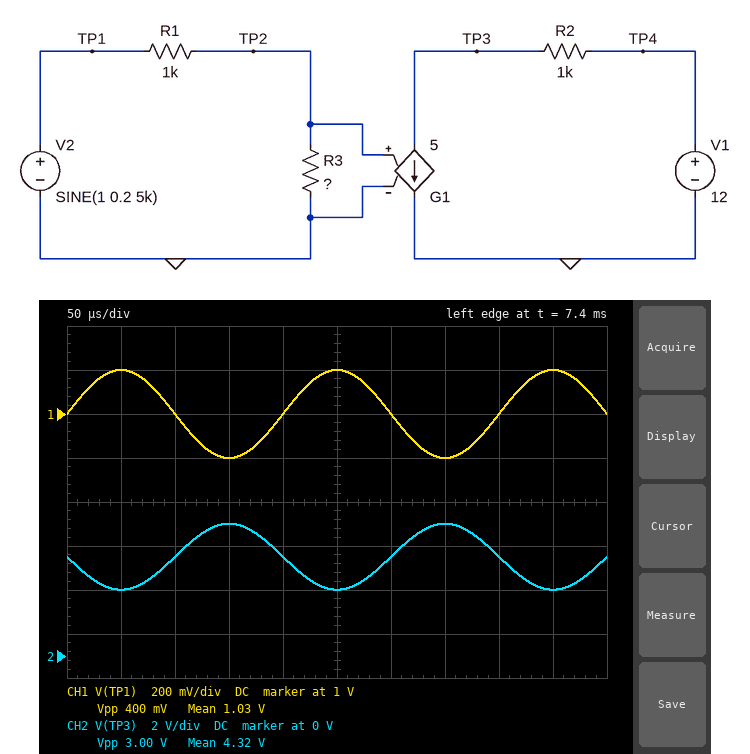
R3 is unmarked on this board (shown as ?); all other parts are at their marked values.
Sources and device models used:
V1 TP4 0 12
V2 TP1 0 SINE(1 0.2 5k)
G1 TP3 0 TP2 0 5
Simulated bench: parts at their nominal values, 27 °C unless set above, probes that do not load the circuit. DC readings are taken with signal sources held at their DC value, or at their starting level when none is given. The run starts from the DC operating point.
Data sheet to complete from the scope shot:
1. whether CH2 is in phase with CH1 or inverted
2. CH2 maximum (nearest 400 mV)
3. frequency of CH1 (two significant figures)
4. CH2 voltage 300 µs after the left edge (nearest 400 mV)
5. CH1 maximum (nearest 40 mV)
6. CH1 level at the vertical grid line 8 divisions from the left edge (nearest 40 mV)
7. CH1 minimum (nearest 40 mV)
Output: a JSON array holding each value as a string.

["inverted", "6.0 V", "5.0 kHz", "4.4 V", "1.20 V", "1.00 V", "800 mV"]
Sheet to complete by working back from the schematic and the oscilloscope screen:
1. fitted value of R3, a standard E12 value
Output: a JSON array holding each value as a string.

["1.5 Ω"]
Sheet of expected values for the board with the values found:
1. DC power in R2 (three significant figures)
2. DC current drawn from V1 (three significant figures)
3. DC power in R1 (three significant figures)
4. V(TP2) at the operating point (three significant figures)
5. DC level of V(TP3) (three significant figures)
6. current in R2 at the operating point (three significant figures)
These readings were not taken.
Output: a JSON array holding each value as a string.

["56.1 mW", "7.49 mA", "997 µW", "1.50 mV", "4.51 V", "7.49 mA"]
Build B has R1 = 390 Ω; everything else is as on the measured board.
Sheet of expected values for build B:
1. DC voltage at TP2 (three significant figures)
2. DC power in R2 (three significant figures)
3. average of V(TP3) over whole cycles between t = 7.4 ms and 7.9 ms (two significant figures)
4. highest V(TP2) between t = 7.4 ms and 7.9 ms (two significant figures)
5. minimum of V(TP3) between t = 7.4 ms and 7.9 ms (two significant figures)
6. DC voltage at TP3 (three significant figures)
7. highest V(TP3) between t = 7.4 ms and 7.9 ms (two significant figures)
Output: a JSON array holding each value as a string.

["3.83 mV", "367 mW", "-7.2 V", "4.6 mV", "-11 V", "-7.16 V", "-3.3 V"]
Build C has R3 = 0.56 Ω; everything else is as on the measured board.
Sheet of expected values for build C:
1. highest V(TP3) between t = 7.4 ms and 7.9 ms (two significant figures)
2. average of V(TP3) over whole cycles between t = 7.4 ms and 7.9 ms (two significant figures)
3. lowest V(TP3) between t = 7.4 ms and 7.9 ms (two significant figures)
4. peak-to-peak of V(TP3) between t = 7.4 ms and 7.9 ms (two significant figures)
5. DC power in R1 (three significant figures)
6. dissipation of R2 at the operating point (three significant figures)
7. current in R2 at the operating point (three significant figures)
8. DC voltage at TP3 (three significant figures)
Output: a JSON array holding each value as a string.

["9.8 V", "9.2 V", "8.6 V", "1.1 V", "999 µW", "7.83 mW", "2.80 mA", "9.20 V"]
